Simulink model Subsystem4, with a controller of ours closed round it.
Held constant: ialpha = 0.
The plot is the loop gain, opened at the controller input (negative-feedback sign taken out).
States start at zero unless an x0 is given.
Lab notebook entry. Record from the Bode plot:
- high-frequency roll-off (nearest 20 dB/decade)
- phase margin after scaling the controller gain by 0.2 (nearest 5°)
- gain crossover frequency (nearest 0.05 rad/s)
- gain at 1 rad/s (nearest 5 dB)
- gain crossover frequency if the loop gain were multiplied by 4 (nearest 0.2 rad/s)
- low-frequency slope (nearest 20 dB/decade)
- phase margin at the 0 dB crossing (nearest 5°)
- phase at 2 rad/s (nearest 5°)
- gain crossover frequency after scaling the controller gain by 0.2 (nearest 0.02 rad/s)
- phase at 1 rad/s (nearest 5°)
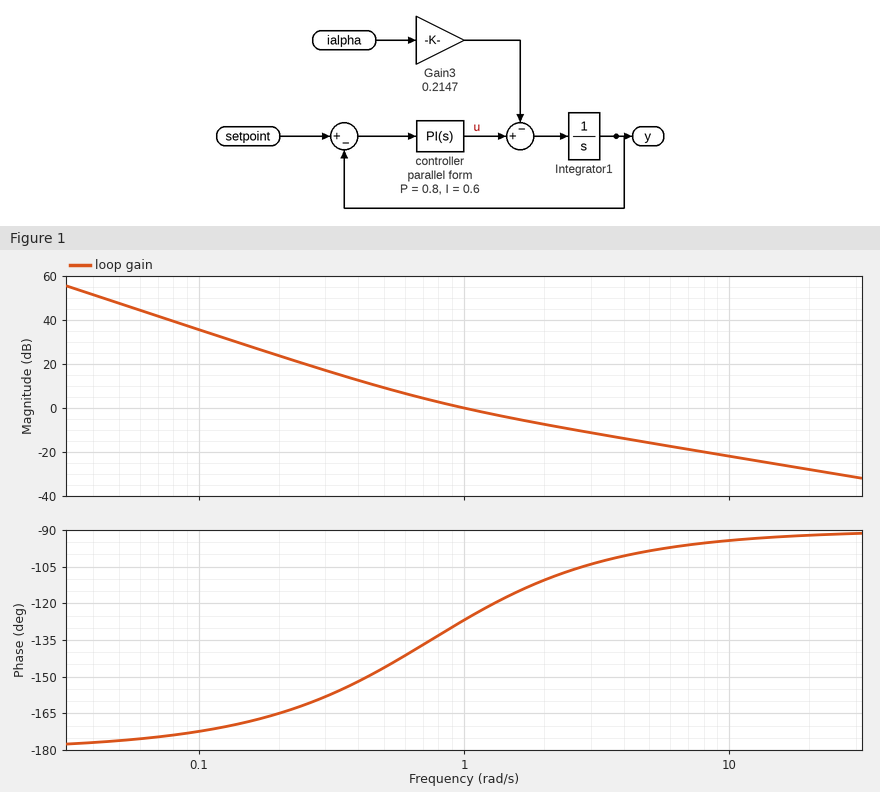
-20 dB/decade
25°
1.00 rad/s
0 dB
3.2 rad/s
-40 dB/decade
55°
-110°
0.36 rad/s
-125°
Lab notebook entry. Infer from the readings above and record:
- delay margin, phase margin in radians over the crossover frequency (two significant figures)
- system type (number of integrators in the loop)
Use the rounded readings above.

0.96 s
2
